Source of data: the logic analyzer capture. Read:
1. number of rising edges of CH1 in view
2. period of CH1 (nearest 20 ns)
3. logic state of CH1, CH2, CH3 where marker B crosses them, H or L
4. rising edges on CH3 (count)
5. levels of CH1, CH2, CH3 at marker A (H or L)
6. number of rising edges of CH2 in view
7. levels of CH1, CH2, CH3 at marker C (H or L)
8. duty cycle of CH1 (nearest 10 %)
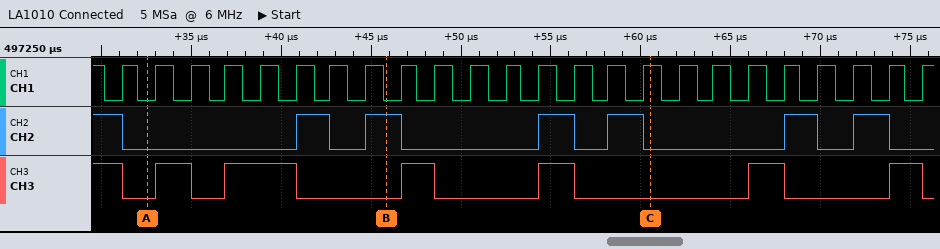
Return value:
24
1940 ns
CH1=L, CH2=H, CH3=L
6
CH1=L, CH2=L, CH3=L
6
CH1=H, CH2=L, CH3=L
50 %
